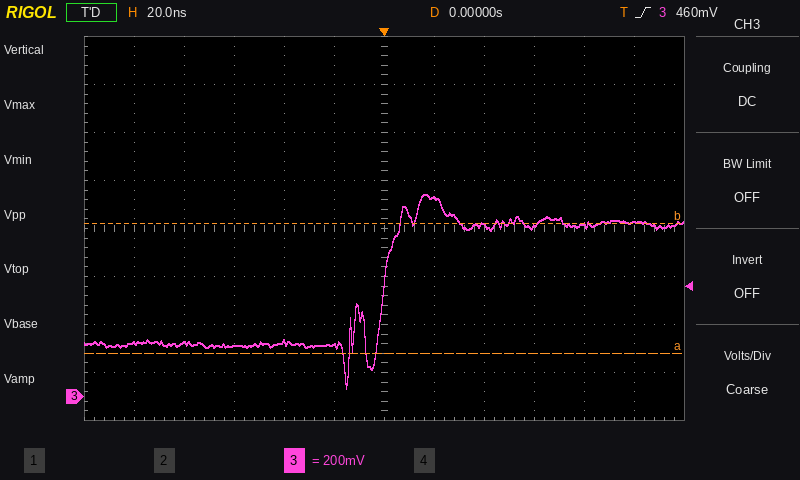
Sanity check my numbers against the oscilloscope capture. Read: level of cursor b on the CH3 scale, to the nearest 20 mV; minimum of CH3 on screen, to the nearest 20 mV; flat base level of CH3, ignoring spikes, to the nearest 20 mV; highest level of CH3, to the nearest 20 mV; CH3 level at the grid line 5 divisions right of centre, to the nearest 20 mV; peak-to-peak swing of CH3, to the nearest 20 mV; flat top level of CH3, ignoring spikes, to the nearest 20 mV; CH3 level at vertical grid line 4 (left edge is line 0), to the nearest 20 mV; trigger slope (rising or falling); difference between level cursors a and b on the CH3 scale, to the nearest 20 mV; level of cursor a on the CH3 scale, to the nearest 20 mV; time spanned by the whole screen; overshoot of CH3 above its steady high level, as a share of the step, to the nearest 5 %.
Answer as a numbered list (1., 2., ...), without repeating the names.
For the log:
1. 720 mV
2. 40 mV
3. 220 mV
4. 840 mV
5. 720 mV
6. 800 mV
7. 720 mV
8. 220 mV
9. rising
10. 540 mV
11. 180 mV
12. 240 ns
13. 25 %
